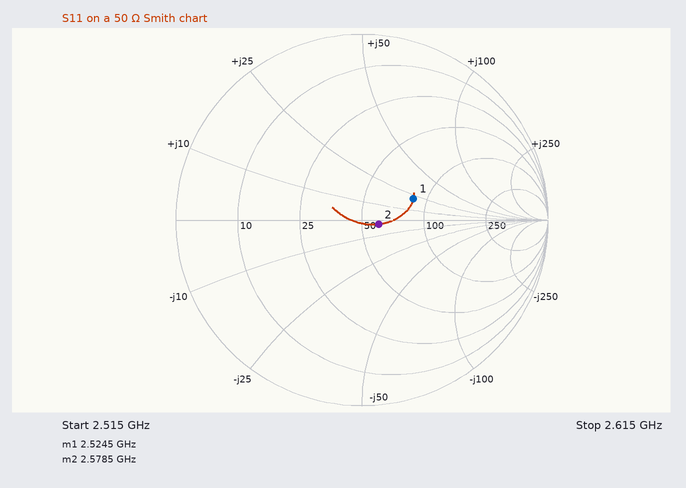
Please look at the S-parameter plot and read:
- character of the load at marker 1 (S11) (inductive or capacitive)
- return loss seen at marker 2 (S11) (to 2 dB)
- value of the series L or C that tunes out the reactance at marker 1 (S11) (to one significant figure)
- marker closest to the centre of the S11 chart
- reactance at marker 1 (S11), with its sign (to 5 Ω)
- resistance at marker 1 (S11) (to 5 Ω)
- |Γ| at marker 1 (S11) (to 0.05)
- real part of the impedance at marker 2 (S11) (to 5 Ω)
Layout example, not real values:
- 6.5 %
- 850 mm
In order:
- inductive
- 20 dB
- 3 pF
- marker 2
- +20 Ω
- 85 Ω
- 0.30
- 60 Ω
